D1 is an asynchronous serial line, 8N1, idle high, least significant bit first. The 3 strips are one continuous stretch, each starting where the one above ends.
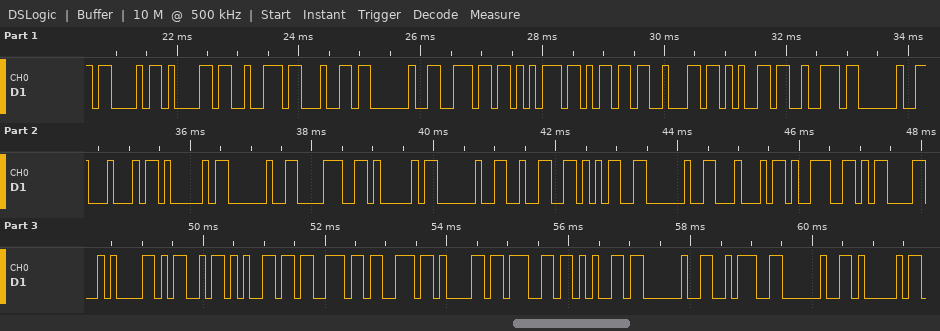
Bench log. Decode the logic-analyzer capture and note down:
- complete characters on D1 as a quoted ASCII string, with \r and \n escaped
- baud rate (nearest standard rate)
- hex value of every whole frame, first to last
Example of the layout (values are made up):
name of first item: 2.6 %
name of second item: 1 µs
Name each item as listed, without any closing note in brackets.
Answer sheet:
complete characters on D1 as a quoted ASCII string, with \r and \n escaped: "Card number DA 8A 25 D9\r\nMessage : A"
baud rate: 9600 baud
hex value of every whole frame, first to last: 0x43 0x61 0x72 0x64 0x20 0x6E 0x75 0x6D 0x62 0x65 0x72 0x20 0x44 0x41 0x20 0x38 0x41 0x20 0x32 0x35 0x20 0x44 0x39 0x0D 0x0A 0x4D 0x65 0x73 0x73 0x61 0x67 0x65 0x20 0x3A 0x20 0x41
